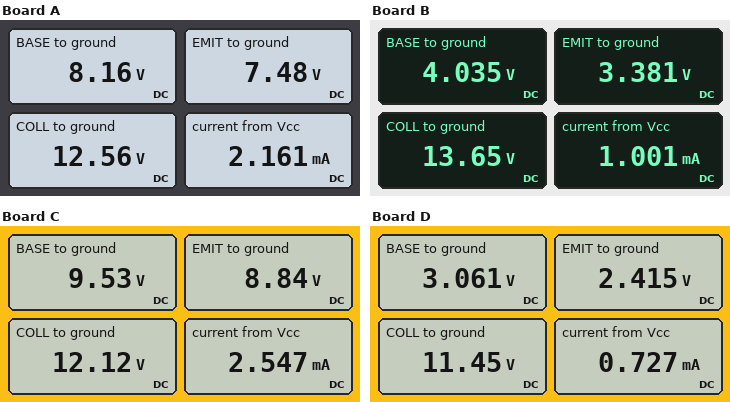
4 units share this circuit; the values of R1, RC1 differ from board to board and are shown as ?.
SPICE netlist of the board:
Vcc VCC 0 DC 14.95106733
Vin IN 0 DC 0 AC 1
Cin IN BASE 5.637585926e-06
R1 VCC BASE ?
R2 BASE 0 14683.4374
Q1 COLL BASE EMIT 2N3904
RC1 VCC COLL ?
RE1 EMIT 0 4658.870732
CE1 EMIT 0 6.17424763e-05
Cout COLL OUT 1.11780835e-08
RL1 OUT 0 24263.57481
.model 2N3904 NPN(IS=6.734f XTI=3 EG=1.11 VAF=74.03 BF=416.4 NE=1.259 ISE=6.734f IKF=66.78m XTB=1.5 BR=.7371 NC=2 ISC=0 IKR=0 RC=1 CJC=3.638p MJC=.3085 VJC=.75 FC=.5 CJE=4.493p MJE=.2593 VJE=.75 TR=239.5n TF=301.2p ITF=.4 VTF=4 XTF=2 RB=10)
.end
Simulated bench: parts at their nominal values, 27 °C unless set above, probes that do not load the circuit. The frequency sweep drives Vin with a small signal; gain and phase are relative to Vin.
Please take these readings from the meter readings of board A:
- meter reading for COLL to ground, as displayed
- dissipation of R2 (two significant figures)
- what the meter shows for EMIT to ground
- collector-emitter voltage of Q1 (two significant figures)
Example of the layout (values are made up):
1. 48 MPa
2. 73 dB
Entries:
1. 12.56 V
2. 4.5 mW
3. 7.48 V
4. 5.1 V
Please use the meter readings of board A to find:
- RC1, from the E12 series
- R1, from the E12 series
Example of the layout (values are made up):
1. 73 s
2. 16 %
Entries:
1. 1.5 kΩ
2. 12 kΩ
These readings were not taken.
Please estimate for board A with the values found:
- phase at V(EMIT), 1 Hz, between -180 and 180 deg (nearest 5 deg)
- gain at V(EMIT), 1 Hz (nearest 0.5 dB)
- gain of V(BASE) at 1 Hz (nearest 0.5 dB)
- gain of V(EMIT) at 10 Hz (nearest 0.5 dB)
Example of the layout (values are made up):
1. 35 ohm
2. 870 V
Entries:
1. 75 deg
2. -13.0 dB
3. -13.0 dB
4. -1.5 dB
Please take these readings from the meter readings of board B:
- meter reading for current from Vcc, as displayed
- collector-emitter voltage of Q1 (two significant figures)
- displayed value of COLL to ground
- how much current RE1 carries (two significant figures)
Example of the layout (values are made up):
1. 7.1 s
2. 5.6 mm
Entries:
1. 1.001 mA
2. 10 V
3. 13.65 V
4. 730 µA
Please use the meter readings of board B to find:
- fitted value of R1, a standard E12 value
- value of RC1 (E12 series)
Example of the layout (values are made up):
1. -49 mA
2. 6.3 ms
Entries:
1. 39 kΩ
2. 1.8 kΩ
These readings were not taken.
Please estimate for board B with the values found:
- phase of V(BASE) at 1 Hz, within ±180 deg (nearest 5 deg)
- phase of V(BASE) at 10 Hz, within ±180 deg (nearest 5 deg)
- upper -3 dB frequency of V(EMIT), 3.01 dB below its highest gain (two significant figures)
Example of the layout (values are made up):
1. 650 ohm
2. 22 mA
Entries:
1. 70 deg
2. 15 deg
3. 81 Hz
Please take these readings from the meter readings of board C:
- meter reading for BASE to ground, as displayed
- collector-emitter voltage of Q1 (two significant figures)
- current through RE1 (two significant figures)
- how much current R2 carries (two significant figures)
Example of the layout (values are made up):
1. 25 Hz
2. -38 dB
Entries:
1. 9.53 V
2. 3.3 V
3. 1.9 mA
4. 650 µA
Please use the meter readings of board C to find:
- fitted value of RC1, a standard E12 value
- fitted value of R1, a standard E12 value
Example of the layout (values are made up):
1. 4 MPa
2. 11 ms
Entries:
1. 1.5 kΩ
2. 8.2 kΩ
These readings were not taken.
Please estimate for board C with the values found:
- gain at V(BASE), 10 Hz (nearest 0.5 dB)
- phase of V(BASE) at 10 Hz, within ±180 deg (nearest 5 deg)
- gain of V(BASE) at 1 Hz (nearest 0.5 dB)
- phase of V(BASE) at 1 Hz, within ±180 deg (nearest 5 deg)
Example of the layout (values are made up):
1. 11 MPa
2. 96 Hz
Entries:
1. -1.5 dB
2. 25 deg
3. -15.0 dB
4. 80 deg
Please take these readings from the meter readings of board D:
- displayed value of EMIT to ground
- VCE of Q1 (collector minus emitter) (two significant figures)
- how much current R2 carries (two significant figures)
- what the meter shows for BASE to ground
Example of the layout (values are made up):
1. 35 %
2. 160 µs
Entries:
1. 2.415 V
2. 9.0 V
3. 210 µA
4. 3.061 V
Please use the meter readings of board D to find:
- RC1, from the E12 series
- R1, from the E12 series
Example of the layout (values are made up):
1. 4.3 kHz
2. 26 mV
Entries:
1. 6.8 kΩ
2. 56 kΩ
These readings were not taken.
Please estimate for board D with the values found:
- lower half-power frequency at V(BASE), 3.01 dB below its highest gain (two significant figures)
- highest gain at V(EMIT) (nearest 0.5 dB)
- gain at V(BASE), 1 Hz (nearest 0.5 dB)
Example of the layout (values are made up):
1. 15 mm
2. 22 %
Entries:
1. 2.7 Hz
2. -1.0 dB
3. -8.5 dB
